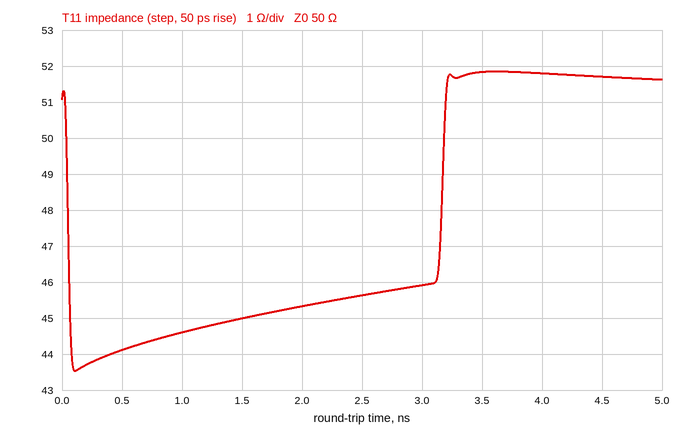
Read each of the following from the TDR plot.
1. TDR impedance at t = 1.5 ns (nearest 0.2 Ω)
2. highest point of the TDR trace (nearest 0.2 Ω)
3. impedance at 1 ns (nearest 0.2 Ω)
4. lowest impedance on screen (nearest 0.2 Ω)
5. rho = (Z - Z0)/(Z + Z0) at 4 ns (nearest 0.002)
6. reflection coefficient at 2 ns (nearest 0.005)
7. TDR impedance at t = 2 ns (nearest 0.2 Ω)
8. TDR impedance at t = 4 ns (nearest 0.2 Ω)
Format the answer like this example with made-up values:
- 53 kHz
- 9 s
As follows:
- 45.0 Ω
- 51.8 Ω
- 44.6 Ω
- 43.6 Ω
- +0.018
- -0.050
- 45.4 Ω
- 51.8 Ω
